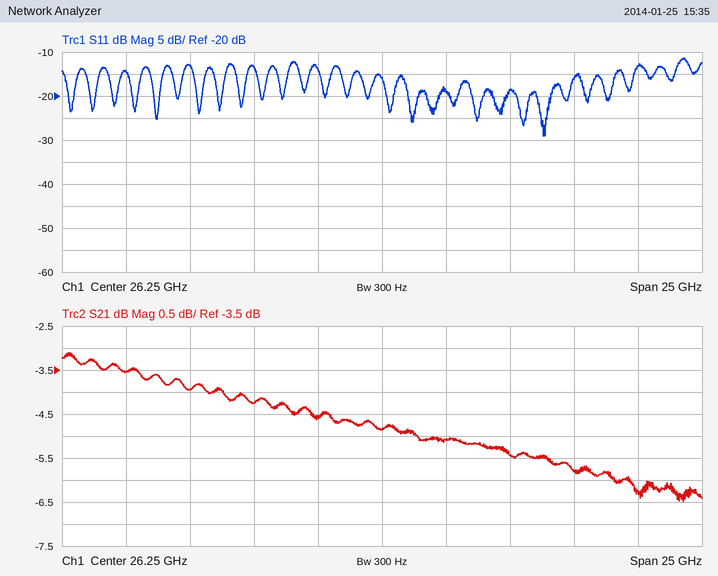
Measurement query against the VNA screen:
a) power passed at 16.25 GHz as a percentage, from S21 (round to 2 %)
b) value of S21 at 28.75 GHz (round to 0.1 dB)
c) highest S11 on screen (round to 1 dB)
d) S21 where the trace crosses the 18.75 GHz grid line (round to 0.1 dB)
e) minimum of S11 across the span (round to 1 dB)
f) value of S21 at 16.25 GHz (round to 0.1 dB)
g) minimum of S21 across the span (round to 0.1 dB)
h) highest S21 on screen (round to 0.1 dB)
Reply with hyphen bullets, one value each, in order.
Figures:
- 44 %
- -5.1 dB
- -11 dB
- -3.9 dB
- -29 dB
- -3.5 dB
- -6.5 dB
- -3.1 dB
